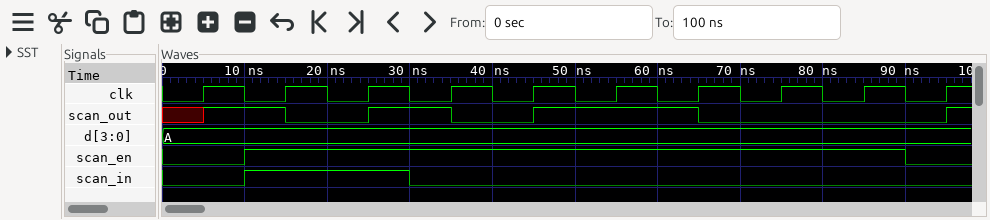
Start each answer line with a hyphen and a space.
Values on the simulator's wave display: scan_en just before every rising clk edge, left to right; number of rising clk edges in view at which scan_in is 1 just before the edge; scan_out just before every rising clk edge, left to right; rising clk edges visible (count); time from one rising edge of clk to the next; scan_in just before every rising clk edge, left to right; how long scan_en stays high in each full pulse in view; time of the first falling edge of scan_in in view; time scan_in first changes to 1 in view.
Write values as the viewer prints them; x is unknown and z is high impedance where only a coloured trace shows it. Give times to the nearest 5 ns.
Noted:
- 0 1 1 1 1 1 1 1 1 0
- 2
- x 1 0 1 0 1 1 0 0 0
- 10
- 10 ns
- 0 1 1 0 0 0 0 0 0 0
- 80 ns
- 30 ns
- 10 ns
